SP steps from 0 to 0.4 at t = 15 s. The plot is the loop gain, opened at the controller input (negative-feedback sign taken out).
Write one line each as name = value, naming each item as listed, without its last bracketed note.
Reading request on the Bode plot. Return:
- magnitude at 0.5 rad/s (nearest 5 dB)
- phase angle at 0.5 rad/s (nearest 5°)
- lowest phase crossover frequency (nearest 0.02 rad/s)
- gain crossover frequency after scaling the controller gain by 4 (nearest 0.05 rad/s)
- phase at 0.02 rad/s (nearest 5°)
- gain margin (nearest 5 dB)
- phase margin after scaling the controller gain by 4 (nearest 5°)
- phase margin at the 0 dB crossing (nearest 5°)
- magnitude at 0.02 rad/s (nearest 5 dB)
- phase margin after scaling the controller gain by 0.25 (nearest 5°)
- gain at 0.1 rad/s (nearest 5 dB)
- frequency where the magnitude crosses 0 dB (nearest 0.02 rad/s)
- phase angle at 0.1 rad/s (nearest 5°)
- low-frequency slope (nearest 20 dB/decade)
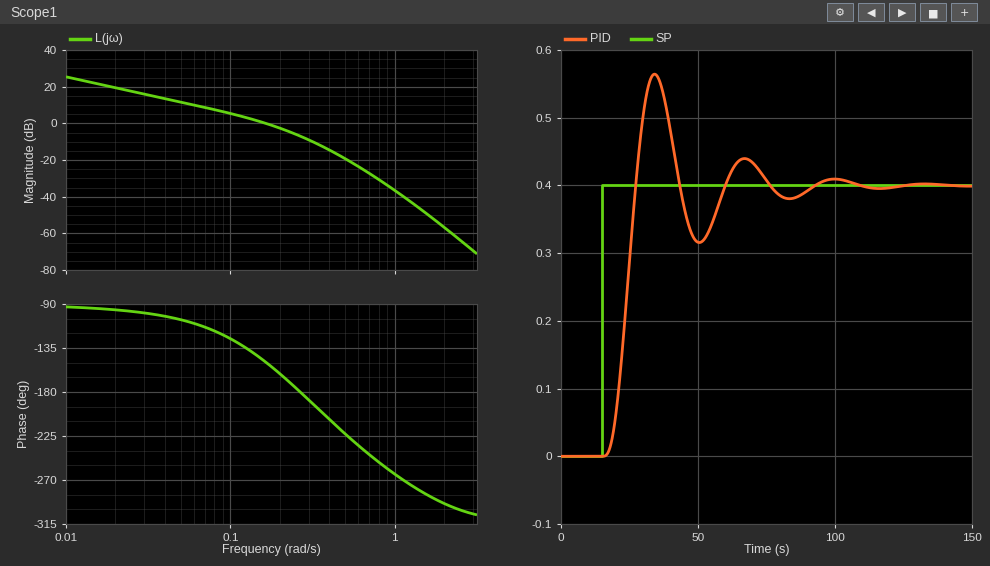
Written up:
magnitude at 0.5 rad/s = -20 dB
phase angle at 0.5 rad/s = -225°
lowest phase crossover frequency = 0.26 rad/s
gain crossover frequency after scaling the controller gain by 4 = 0.35 rad/s
phase at 0.02 rad/s = -95°
gain margin = 5 dB
phase margin after scaling the controller gain by 4 = -20°
phase margin at the 0 dB crossing = 30°
magnitude at 0.02 rad/s = 20 dB
phase margin after scaling the controller gain by 0.25 = 75°
gain at 0.1 rad/s = 5 dB
frequency where the magnitude crosses 0 dB = 0.16 rad/s
phase angle at 0.1 rad/s = -125°
low-frequency slope = -20 dB/decade
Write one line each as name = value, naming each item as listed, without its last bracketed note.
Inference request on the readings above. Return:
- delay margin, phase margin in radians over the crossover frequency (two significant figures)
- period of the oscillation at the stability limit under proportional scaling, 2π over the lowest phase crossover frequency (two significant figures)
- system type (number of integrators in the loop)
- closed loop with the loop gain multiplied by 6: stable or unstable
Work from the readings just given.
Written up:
delay margin, phase margin in radians over the crossover frequency = 3.3 s
period of the oscillation at the stability limit under proportional scaling, 2π over the lowest phase crossover frequency = 24 s
system type = 1
closed loop with the loop gain multiplied by 6: stable or unstable = unstable
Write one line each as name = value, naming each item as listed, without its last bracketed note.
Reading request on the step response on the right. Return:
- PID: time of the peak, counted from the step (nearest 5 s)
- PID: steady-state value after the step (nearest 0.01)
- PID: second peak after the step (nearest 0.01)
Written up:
PID: time of the peak, counted from the step = 20 s
PID: steady-state value after the step = 0.40
PID: second peak after the step = 0.44
